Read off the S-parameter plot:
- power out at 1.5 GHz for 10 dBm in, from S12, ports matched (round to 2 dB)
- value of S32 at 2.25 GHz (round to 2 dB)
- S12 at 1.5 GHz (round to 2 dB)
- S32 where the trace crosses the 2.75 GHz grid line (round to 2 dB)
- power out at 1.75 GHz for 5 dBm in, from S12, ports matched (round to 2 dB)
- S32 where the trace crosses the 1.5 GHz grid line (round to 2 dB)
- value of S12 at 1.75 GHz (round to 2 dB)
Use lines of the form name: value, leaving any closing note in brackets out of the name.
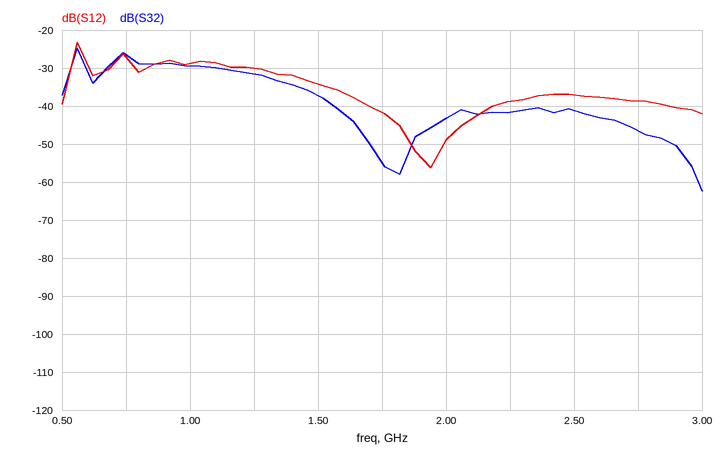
power out at 1.5 GHz for 10 dBm in, from S12, ports matched: -24 dBm
value of S32 at 2.25 GHz: -42 dB
S12 at 1.5 GHz: -34 dB
S32 where the trace crosses the 2.75 GHz grid line: -46 dB
power out at 1.75 GHz for 5 dBm in, from S12, ports matched: -36 dBm
S32 where the trace crosses the 1.5 GHz grid line: -38 dB
value of S12 at 1.75 GHz: -42 dB
